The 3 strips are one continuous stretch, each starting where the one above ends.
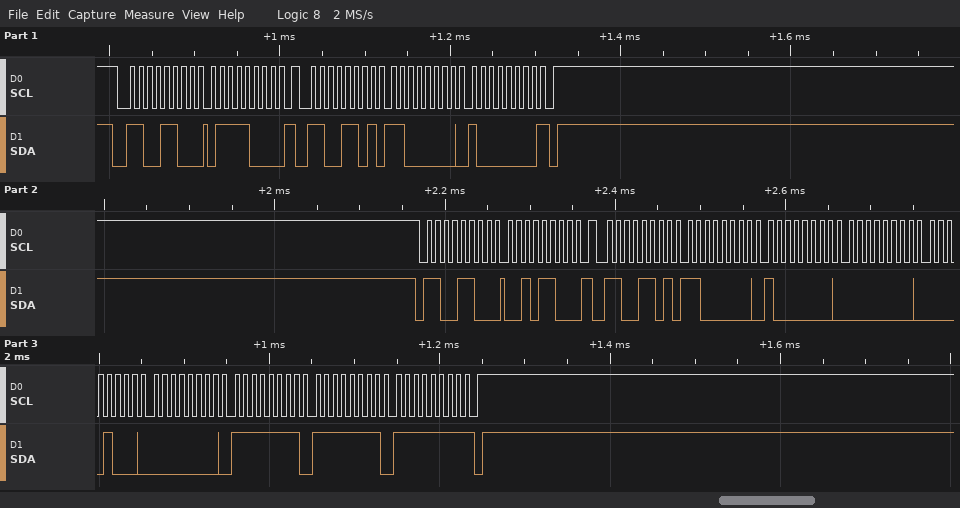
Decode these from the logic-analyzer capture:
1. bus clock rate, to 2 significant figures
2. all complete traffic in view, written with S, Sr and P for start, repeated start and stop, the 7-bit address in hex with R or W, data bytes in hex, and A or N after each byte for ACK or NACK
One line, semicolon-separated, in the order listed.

100 kHz; S 66W A 78 A Sr 66R A C0 A 80 N P S 66W A 2C A Sr 66R A C0 A 80 A 00 A 08 A 00 A FF A FF A FF N P
